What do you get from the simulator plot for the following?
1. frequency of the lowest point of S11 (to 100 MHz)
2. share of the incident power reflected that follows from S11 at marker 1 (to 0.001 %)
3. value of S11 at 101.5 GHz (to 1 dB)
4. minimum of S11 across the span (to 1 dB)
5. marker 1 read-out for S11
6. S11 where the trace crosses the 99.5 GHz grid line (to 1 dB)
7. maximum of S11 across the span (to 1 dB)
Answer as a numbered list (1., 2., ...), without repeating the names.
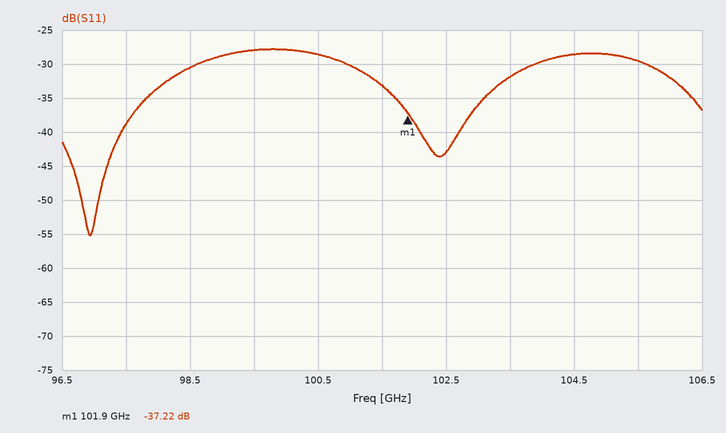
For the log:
1. 96.9 GHz
2. 0.019 %
3. -33 dB
4. -55 dB
5. -37.22 dB
6. -28 dB
7. -28 dB
